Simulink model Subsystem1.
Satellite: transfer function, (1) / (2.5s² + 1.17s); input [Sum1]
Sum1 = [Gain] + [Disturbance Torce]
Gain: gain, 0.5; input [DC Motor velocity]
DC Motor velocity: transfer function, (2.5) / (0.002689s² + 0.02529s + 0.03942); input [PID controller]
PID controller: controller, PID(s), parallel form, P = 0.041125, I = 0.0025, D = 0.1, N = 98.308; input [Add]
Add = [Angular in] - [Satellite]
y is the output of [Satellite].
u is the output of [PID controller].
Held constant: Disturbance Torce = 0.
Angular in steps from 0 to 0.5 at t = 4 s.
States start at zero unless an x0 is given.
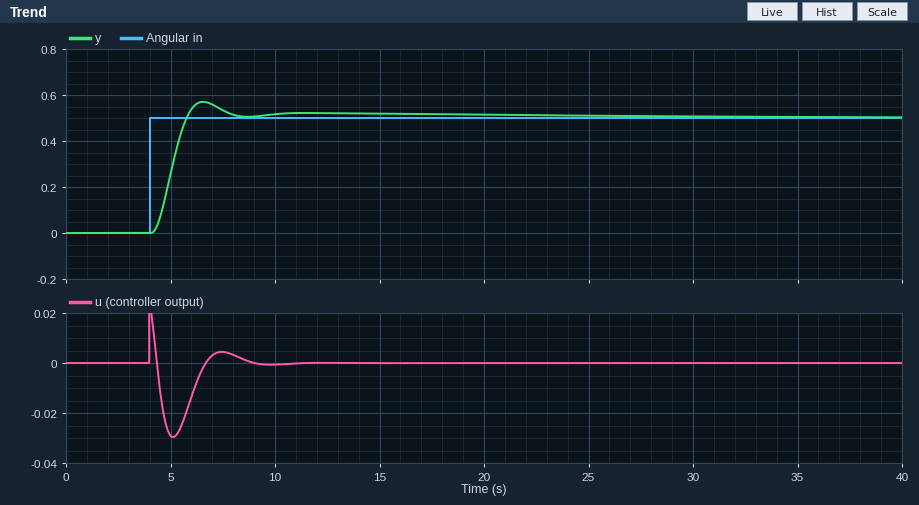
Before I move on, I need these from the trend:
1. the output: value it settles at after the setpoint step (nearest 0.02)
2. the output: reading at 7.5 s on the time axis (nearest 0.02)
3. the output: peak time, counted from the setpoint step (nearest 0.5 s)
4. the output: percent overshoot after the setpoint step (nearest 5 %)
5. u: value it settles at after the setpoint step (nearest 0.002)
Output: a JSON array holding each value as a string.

["0.50", "0.54", "2.5 s", "15 %", "0.000"]
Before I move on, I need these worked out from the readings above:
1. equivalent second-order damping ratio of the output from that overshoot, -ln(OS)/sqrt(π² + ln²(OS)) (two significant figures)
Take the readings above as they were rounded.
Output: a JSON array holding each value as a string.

["0.52"]
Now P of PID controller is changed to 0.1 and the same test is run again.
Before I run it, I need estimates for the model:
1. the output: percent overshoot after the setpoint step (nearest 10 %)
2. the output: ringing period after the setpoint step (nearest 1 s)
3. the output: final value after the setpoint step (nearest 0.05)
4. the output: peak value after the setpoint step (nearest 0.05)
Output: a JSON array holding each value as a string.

["50 %", "5 s", "0.50", "0.75"]
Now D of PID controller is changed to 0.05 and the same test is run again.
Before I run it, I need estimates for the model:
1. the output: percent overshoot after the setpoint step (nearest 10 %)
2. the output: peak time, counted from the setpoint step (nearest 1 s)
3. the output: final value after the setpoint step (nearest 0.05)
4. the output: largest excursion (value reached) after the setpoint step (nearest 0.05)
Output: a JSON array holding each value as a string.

["30 %", "4 s", "0.50", "0.65"]
